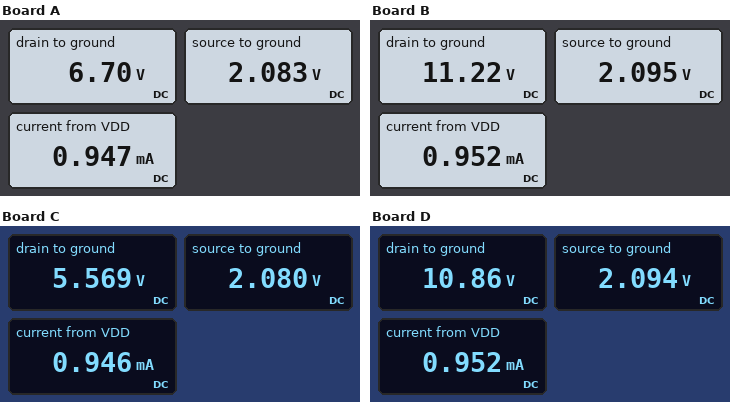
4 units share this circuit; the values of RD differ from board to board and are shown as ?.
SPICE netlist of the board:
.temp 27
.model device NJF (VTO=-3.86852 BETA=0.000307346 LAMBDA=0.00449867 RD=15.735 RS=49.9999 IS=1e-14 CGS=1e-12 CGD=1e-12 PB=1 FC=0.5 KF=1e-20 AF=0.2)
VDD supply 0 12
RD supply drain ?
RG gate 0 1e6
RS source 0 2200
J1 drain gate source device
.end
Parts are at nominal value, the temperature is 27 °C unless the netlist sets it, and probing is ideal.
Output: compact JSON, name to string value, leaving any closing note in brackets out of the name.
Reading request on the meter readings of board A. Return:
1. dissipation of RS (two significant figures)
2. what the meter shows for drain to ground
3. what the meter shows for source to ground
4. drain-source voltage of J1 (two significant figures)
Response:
{"dissipation of RS": "2.0 mW", "what the meter shows for drain to ground": "6.70 V", "what the meter shows for source to ground": "2.083 V", "drain-source voltage of J1": "4.6 V"}
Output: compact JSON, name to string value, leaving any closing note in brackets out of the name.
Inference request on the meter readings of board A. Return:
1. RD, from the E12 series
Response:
{"RD, from the E12 series": "5.6 kΩ"}
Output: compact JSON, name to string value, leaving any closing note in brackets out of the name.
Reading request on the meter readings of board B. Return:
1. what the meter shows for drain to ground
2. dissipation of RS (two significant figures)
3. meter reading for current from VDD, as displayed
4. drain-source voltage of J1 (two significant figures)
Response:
{"what the meter shows for drain to ground": "11.22 V", "dissipation of RS": "2.0 mW", "meter reading for current from VDD, as displayed": "0.952 mA", "drain-source voltage of J1": "9.1 V"}
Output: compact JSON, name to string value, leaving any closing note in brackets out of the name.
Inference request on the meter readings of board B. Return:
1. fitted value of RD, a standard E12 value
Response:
{"fitted value of RD, a standard E12 value": "820 Ω"}
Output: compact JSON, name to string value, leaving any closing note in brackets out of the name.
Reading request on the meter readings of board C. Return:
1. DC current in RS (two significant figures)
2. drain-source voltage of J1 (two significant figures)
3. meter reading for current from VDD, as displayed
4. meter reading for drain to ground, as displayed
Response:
{"DC current in RS": "950 µA", "drain-source voltage of J1": "3.5 V", "meter reading for current from VDD, as displayed": "0.946 mA", "meter reading for drain to ground, as displayed": "5.569 V"}
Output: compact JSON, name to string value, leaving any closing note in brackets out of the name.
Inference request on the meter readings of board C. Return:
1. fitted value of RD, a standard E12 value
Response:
{"fitted value of RD, a standard E12 value": "6.8 kΩ"}
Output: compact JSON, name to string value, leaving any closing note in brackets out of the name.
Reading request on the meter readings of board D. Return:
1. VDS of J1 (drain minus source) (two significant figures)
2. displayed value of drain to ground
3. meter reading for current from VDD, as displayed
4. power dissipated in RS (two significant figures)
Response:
{"VDS of J1 (drain minus source)": "8.8 V", "displayed value of drain to ground": "10.86 V", "meter reading for current from VDD, as displayed": "0.952 mA", "power dissipated in RS": "2.0 mW"}
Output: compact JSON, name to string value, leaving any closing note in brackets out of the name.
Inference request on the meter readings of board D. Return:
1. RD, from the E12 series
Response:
{"RD, from the E12 series": "1.2 kΩ"}
